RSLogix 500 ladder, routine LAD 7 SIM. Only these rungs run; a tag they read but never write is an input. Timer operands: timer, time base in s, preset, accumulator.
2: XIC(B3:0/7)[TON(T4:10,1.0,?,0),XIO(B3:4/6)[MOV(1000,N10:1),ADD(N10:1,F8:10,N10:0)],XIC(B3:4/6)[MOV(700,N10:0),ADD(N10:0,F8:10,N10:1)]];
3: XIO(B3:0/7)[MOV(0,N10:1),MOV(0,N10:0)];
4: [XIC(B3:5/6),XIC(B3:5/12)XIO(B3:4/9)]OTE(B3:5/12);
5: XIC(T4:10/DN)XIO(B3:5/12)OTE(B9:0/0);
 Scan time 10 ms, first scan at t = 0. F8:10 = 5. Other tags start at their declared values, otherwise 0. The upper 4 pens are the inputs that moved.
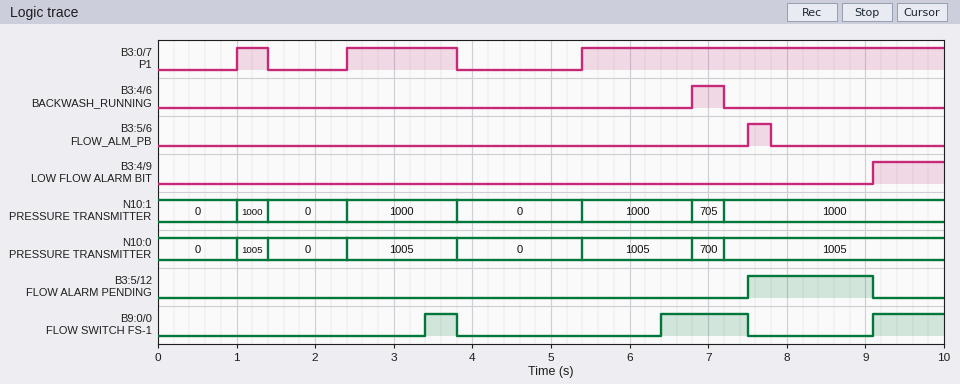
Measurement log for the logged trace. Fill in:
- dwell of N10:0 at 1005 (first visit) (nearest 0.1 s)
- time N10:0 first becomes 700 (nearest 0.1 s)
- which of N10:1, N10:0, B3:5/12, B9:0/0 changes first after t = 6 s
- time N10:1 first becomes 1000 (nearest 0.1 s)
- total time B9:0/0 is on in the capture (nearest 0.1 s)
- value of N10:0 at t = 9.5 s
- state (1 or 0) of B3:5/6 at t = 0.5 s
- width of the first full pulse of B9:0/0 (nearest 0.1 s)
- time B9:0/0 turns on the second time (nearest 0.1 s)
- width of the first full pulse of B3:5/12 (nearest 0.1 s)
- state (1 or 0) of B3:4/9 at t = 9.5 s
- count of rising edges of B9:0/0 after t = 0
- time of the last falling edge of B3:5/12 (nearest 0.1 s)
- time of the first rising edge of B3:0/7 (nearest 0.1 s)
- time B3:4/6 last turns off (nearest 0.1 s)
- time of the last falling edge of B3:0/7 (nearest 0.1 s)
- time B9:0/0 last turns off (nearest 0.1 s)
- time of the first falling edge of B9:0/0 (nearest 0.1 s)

0.4 s
6.8 s
B9:0/0
1.0 s
2.4 s
1005
0
0.4 s
6.4 s
1.6 s
1
3
9.1 s
1.0 s
7.2 s
3.8 s
7.5 s
3.8 s
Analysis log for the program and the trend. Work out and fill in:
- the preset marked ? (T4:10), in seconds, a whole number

1 s
